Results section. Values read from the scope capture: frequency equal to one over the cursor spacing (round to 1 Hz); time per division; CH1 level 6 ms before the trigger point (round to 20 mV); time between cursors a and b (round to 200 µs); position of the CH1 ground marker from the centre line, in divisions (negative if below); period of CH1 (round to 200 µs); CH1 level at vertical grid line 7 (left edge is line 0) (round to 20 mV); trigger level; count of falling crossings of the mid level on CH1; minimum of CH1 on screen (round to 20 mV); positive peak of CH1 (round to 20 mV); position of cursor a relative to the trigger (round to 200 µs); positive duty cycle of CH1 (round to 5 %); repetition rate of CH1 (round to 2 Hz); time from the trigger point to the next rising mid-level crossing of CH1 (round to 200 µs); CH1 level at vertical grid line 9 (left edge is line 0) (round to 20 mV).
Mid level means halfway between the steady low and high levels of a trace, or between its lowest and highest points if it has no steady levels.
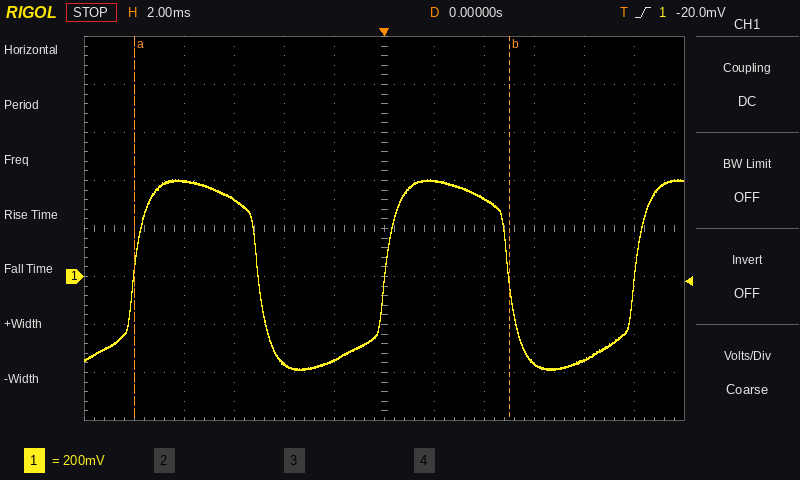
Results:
67 Hz
2 ms
320 mV
15.0 ms
-1.0 div
10.0 ms
400 mV
-20.0 mV
2
-380 mV
400 mV
-10.0 ms
50 %
100 Hz
10.0 ms
-360 mV
